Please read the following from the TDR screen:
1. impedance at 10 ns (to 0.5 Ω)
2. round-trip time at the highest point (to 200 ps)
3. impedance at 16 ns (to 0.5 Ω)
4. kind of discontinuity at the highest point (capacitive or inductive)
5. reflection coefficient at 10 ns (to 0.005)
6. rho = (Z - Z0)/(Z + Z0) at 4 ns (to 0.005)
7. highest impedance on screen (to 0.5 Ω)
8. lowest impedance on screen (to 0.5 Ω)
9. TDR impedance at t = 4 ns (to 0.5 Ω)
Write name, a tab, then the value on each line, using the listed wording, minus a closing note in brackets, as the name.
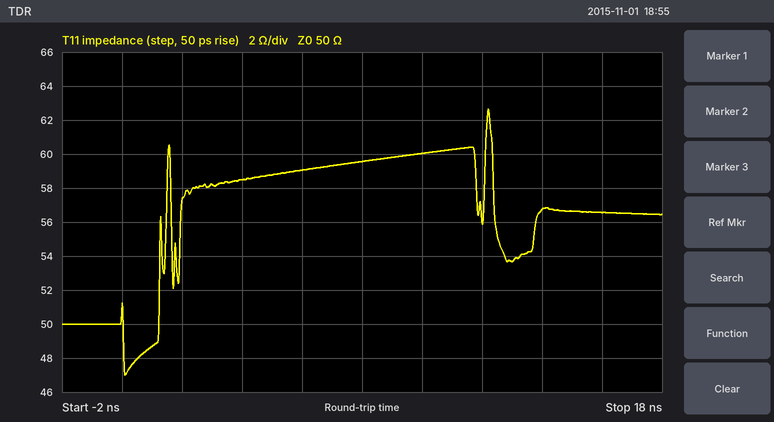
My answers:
impedance at 10 ns	60.0 Ω
round-trip time at the highest point	12.2 ns
impedance at 16 ns	56.5 Ω
kind of discontinuity at the highest point	inductive
reflection coefficient at 10 ns	+0.090
rho = (Z - Z0)/(Z + Z0) at 4 ns	+0.080
highest impedance on screen	62.5 Ω
lowest impedance on screen	47.0 Ω
TDR impedance at t = 4 ns	58.5 Ω
